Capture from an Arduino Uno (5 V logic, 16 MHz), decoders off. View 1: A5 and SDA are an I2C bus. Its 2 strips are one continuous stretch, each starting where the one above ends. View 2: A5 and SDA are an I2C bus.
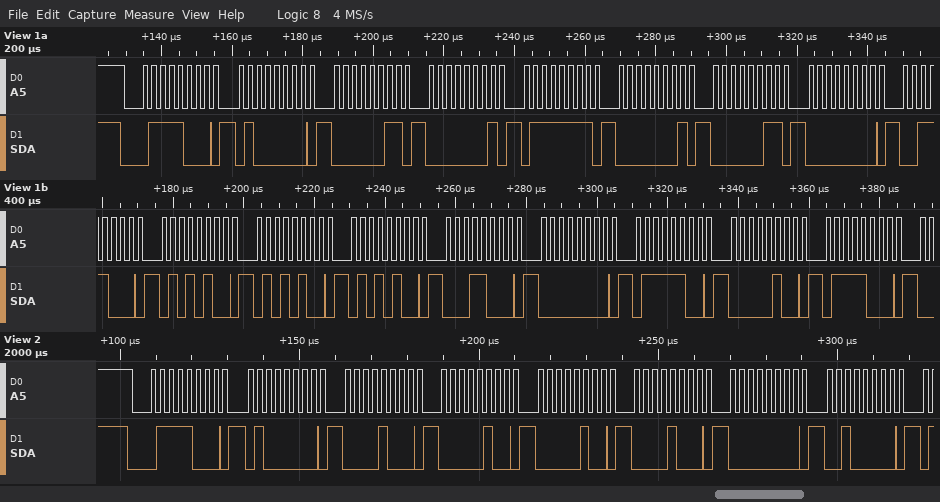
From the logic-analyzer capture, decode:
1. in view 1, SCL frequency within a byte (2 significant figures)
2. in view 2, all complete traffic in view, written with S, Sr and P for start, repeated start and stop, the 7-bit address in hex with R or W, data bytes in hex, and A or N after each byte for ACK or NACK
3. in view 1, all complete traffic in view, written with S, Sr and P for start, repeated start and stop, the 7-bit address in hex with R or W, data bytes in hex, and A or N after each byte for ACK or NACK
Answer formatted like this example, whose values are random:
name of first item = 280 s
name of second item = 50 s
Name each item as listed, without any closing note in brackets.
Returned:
in view 1, SCL frequency within a byte = 400 kHz
in view 2, all complete traffic in view, written with S, Sr and P for start, repeated start and stop, the 7-bit address in hex with R or W, data bytes in hex, and A or N after each byte for ACK or NACK = S 3CW A 40 A 08 A 04 A 04 A 08 A 00 A 20 A
in view 1, all complete traffic in view, written with S, Sr and P for start, repeated start and stop, the 7-bit address in hex with R or W, data bytes in hex, and A or N after each byte for ACK or NACK = S 3CW A 40 A 03 A 01 A 7F A 01 A 03 A 00 A 38 A 54 A 54 A 54 A 18 A 00 A 7C A 04 A 78 A
